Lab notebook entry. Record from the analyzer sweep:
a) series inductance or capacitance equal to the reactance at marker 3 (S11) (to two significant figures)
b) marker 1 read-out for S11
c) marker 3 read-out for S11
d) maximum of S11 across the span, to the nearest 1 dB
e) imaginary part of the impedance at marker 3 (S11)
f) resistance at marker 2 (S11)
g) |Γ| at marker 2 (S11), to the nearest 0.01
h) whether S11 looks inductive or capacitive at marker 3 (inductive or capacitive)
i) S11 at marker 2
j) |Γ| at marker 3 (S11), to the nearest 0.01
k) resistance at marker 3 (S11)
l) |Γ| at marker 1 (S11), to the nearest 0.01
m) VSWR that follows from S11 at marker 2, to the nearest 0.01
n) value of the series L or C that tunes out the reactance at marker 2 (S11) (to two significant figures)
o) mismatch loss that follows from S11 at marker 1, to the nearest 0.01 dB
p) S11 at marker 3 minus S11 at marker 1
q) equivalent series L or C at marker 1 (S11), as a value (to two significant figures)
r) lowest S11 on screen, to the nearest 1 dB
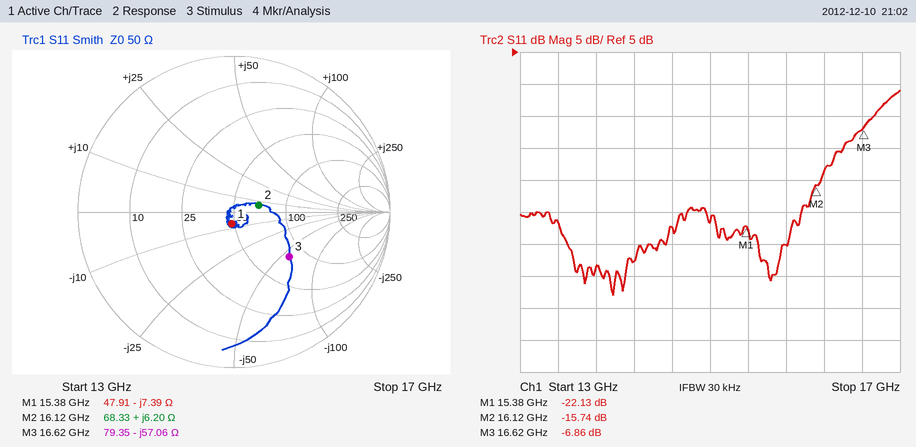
170 fF
-22.13 dB
-6.86 dB
-1 dB
-57.06 Ω
68.33 Ω
0.16
capacitive
-15.74 dB
0.45
79.35 Ω
0.08
1.39
1.6 pF
0.03 dB
15.27 dB
1.4 pF
-33 dB
